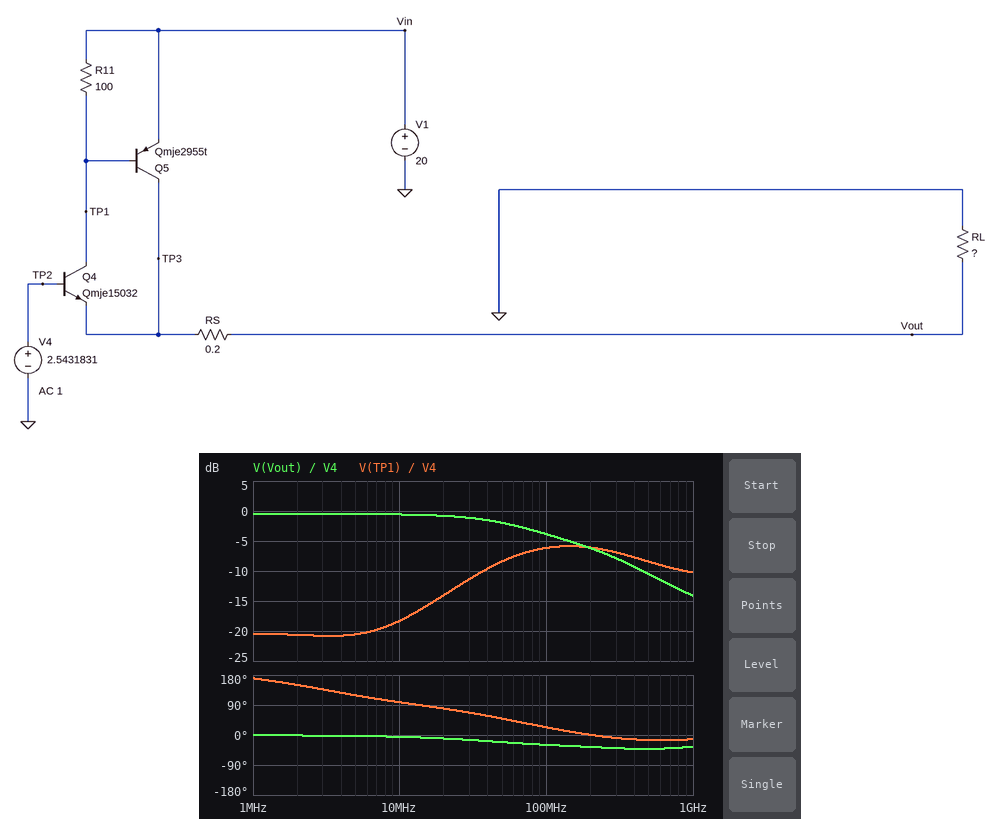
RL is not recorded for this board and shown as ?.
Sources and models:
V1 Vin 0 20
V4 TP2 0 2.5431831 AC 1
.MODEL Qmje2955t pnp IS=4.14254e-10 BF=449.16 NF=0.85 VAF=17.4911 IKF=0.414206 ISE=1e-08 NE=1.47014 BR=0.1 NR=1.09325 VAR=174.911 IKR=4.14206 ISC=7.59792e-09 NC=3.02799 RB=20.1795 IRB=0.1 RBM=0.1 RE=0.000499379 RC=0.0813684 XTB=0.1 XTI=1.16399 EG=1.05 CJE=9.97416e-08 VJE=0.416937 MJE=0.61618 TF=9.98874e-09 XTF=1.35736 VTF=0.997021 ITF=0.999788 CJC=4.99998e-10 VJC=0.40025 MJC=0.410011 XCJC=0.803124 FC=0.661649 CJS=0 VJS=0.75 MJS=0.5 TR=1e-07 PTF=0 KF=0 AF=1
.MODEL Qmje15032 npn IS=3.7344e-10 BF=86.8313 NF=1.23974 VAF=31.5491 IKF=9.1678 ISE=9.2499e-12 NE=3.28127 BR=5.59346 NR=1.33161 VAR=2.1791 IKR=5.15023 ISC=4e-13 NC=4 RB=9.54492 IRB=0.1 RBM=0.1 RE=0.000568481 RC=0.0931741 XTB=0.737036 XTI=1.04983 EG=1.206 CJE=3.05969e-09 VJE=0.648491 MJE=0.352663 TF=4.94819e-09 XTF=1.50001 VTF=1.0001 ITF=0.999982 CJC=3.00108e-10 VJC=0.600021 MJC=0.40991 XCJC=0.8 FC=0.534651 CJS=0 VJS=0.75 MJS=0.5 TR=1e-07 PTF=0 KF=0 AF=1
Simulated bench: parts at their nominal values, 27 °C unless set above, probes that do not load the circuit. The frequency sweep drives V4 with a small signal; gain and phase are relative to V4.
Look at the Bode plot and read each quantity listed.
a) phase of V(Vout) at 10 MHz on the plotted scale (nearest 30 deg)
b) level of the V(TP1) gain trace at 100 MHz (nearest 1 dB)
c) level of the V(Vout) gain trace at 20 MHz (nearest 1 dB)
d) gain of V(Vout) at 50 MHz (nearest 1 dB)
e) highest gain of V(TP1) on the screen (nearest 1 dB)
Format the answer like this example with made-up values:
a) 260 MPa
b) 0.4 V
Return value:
a) 0 deg
b) -6 dB
c) -1 dB
d) -2 dB
e) -6 dB
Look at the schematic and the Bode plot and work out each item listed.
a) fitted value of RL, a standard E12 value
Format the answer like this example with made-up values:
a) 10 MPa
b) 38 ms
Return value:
a) 180 Ω
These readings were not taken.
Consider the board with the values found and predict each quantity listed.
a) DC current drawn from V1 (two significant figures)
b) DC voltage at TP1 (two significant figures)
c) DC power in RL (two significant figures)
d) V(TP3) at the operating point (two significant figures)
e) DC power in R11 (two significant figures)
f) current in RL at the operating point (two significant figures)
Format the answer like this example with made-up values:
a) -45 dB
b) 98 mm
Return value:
a) 11 mA
b) 20 V
c) 23 mW
d) 2.0 V
e) 1.3 mW
f) 11 mA
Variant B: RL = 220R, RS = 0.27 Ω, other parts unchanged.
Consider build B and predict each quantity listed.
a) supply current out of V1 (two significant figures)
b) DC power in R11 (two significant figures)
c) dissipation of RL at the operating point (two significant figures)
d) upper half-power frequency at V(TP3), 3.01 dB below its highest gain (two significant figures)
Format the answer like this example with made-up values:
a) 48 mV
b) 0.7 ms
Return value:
a) 9.2 mA
b) 1.2 mW
c) 19 mW
d) 78 MHz
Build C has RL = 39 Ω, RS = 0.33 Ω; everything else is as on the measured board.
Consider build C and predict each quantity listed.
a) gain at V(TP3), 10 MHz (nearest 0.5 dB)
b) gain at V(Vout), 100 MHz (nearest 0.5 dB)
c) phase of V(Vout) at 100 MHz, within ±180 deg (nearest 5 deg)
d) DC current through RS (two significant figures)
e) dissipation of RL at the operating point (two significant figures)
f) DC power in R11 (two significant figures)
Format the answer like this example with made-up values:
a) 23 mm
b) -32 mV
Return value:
a) -2.0 dB
b) -5.0 dB
c) -25 deg
d) 52 mA
e) 100 mW
f) 1.6 mW
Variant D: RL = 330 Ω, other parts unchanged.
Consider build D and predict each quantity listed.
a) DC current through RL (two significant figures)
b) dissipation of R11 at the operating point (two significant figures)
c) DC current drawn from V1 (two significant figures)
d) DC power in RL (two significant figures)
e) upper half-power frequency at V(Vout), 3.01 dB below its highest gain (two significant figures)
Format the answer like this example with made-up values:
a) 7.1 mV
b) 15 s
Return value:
a) 6.2 mA
b) 1.1 mW
c) 6.1 mA
d) 13 mW
e) 80 MHz
